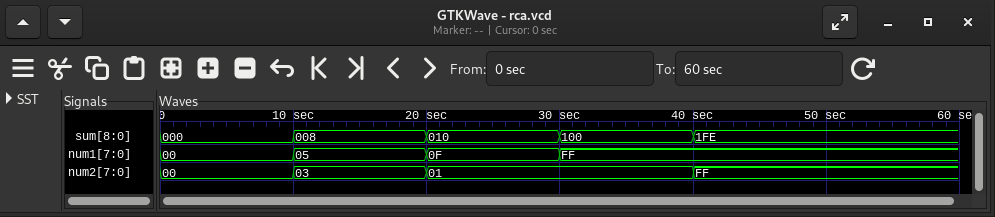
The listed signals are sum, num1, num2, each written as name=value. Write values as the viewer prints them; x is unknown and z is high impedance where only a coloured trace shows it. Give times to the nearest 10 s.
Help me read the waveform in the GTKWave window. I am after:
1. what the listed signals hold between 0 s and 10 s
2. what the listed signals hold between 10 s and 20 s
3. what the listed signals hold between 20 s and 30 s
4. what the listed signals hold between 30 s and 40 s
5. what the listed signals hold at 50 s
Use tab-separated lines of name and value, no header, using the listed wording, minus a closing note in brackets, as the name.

what the listed signals hold between 0 s and 10 s	sum=000, num1=00, num2=00
what the listed signals hold between 10 s and 20 s	sum=008, num1=05, num2=03
what the listed signals hold between 20 s and 30 s	sum=010, num1=0F, num2=01
what the listed signals hold between 30 s and 40 s	sum=100, num1=FF, num2=01
what the listed signals hold at 50 s	sum=1FE, num1=FF, num2=FF
